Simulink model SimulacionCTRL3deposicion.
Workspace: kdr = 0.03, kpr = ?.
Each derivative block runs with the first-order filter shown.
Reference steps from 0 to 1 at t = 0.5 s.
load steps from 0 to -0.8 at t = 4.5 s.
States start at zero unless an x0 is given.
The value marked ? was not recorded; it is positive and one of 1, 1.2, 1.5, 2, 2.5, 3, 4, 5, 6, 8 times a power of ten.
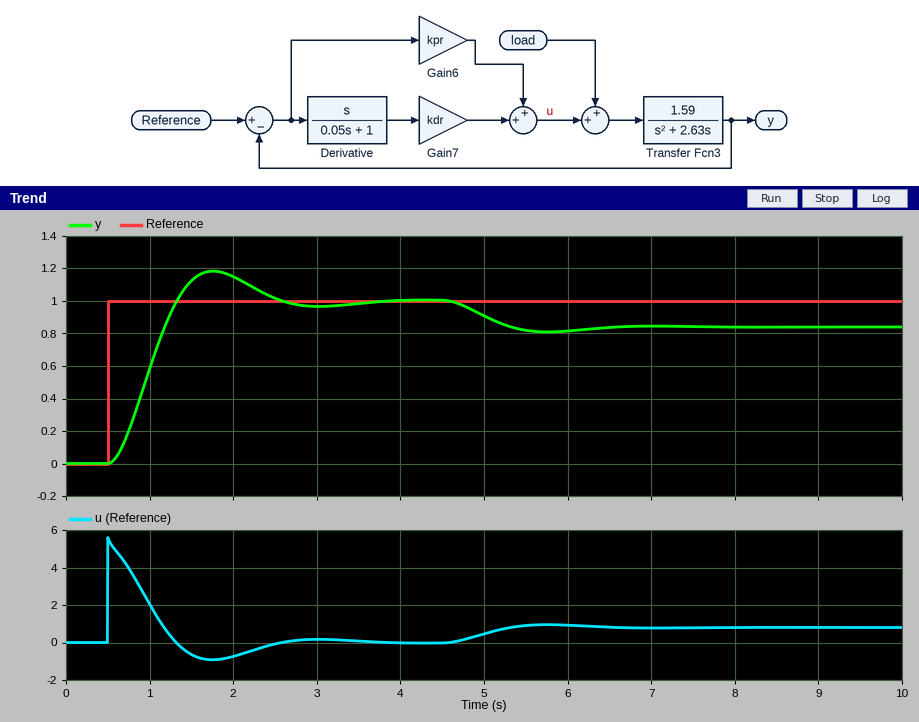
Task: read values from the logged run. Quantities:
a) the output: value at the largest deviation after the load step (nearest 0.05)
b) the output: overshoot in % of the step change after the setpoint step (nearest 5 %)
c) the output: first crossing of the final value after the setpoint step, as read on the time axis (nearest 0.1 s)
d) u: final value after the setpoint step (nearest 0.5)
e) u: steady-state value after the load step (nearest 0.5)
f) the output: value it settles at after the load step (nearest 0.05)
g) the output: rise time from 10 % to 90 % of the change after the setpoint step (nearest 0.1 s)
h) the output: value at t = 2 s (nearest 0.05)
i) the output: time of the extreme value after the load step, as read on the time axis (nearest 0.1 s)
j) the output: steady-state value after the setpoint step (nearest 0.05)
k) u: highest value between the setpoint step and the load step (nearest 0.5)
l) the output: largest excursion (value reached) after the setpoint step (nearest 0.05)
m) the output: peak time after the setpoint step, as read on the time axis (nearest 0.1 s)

0.80
20 %
1.3 s
0.0
1.0
0.85
0.6 s
1.15
5.8 s
1.00
5.5
1.20
1.8 s
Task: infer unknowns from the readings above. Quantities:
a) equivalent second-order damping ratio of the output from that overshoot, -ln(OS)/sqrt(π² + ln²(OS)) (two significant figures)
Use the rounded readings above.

0.46
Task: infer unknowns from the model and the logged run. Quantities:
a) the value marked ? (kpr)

5
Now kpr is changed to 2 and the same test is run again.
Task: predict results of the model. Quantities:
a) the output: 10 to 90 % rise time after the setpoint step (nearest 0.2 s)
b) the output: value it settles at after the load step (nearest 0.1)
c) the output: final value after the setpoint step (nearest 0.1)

1.2 s
0.6
1.0
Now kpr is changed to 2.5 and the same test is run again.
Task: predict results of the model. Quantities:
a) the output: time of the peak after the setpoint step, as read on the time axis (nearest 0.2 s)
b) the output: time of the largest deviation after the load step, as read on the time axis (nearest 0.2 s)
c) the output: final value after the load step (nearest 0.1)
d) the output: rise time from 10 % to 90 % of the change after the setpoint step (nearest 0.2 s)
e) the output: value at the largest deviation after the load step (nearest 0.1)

2.6 s
6.6 s
0.7
1.0 s
0.7
